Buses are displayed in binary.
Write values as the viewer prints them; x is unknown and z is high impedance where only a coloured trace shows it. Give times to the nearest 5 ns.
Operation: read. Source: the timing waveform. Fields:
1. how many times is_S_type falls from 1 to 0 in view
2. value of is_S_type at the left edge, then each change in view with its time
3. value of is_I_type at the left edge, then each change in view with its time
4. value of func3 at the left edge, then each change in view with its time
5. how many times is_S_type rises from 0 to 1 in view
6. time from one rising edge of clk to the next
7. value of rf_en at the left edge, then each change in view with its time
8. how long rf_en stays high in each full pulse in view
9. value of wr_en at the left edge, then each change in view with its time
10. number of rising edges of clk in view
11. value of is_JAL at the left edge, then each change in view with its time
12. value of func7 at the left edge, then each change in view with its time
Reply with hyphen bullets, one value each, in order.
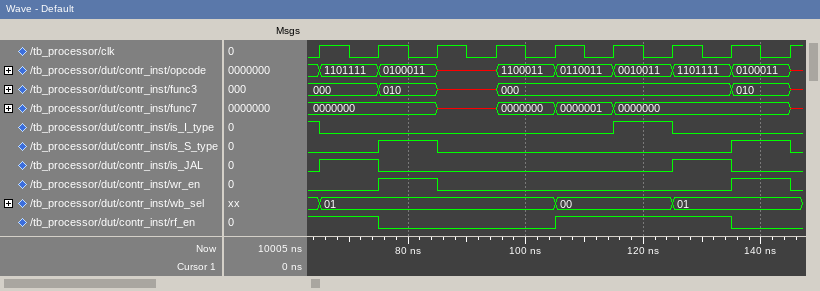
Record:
- 2
- 0, 1 at 75 ns, 0 at 85 ns, 1 at 135 ns, 0 at 145 ns
- 1, 0 at 65 ns, 1 at 115 ns, 0 at 125 ns
- 000, 010 at 75 ns, x at 85 ns, 000 at 95 ns, 010 at 135 ns, x at 145 ns
- 2
- 10 ns
- 1, 0 at 75 ns, 1 at 105 ns, 0 at 135 ns
- 30 ns
- 0, 1 at 75 ns, 0 at 85 ns, 1 at 135 ns, 0 at 145 ns
- 9
- 0, 1 at 65 ns, 0 at 75 ns, 1 at 125 ns, 0 at 135 ns
- 0000000, x at 85 ns, 0000000 at 95 ns, 0000001 at 105 ns, 0000000 at 115 ns, x at 145 ns
